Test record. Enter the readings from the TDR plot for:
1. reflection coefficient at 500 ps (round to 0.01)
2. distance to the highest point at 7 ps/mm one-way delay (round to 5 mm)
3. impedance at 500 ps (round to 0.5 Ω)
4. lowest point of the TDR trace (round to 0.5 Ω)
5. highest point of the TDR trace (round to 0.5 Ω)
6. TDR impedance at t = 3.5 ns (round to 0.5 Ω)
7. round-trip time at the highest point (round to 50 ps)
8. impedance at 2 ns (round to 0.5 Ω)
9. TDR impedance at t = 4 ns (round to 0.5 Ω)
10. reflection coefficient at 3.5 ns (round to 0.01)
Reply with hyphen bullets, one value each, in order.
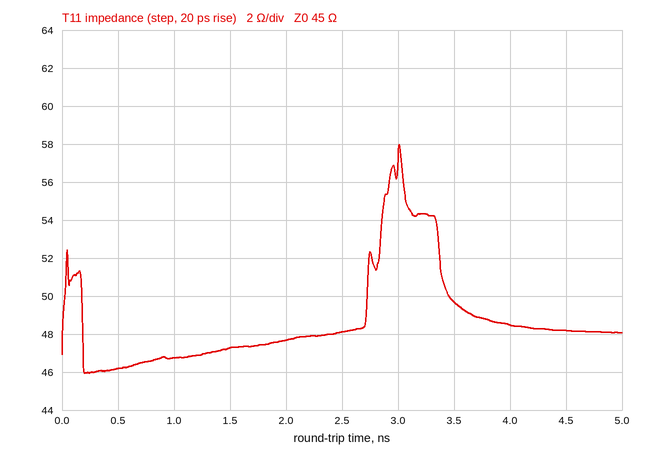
- +0.01
- 215 mm
- 46.0 Ω
- 46.0 Ω
- 58.0 Ω
- 49.5 Ω
- 3.00 ns
- 47.5 Ω
- 48.5 Ω
- +0.05
